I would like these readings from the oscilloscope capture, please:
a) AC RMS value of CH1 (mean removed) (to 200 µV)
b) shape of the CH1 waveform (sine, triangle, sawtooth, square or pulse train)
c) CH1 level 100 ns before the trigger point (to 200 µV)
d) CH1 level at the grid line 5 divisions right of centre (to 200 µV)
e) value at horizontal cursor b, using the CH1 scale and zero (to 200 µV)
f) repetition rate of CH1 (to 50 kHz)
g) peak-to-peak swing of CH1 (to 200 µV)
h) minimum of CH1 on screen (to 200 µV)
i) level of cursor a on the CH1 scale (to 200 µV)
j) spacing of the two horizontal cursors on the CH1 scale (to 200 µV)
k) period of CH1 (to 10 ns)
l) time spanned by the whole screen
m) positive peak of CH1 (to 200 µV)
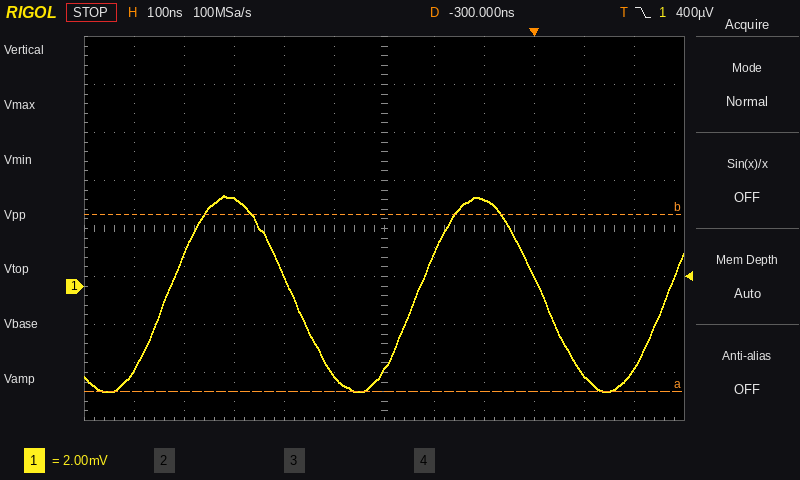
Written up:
2.8 mV
sine
3.6 mV
-3.4 mV
3.0 mV
2.00 MHz
8.2 mV
-4.4 mV
-4.4 mV
7.4 mV
500 ns
1.2 µs
3.8 mV
